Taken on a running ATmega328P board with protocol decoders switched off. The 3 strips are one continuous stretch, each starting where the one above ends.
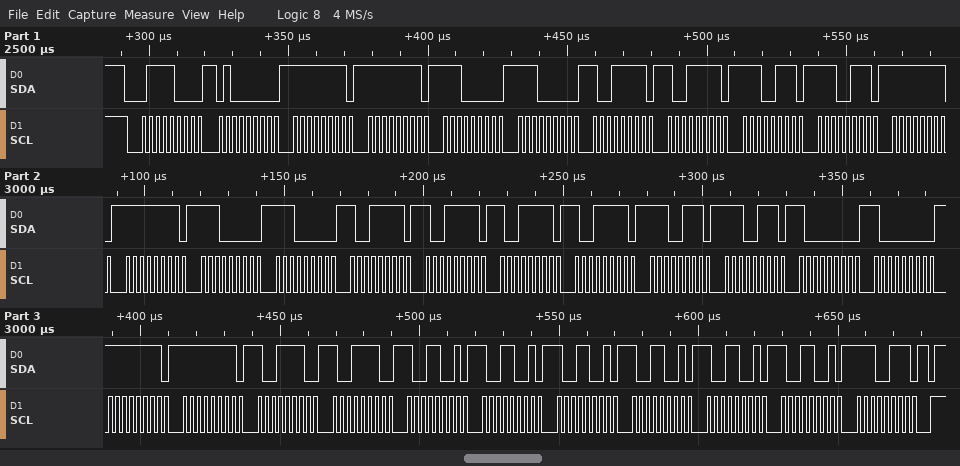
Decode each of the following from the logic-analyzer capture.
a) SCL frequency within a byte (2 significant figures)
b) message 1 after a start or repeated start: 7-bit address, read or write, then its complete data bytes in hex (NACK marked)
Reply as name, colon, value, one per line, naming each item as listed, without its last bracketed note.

SCL frequency within a byte: 400 kHz
message 1 after a start or repeated start: 7-bit address, read or write, then its complete data bytes in hex: 0x3C write: 40 FF FF E0 E0 9F 9F E7 E7 FF FF E0 E0 9F 9F 9F 9F E7 E7 80 80 FF FF 9E 9E 99 99 99 99 99 99 E7
